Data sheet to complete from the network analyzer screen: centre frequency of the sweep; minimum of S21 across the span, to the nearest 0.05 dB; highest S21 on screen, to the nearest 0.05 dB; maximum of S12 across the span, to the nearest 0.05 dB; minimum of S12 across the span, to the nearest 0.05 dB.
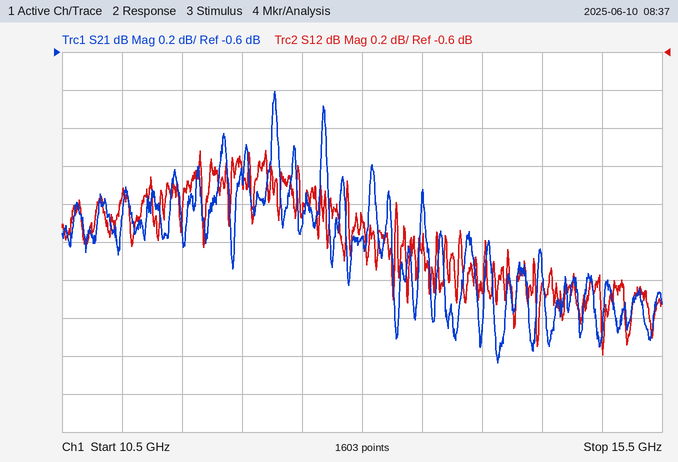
13 GHz
-2.25 dB
-0.80 dB
-1.10 dB
-2.20 dB
